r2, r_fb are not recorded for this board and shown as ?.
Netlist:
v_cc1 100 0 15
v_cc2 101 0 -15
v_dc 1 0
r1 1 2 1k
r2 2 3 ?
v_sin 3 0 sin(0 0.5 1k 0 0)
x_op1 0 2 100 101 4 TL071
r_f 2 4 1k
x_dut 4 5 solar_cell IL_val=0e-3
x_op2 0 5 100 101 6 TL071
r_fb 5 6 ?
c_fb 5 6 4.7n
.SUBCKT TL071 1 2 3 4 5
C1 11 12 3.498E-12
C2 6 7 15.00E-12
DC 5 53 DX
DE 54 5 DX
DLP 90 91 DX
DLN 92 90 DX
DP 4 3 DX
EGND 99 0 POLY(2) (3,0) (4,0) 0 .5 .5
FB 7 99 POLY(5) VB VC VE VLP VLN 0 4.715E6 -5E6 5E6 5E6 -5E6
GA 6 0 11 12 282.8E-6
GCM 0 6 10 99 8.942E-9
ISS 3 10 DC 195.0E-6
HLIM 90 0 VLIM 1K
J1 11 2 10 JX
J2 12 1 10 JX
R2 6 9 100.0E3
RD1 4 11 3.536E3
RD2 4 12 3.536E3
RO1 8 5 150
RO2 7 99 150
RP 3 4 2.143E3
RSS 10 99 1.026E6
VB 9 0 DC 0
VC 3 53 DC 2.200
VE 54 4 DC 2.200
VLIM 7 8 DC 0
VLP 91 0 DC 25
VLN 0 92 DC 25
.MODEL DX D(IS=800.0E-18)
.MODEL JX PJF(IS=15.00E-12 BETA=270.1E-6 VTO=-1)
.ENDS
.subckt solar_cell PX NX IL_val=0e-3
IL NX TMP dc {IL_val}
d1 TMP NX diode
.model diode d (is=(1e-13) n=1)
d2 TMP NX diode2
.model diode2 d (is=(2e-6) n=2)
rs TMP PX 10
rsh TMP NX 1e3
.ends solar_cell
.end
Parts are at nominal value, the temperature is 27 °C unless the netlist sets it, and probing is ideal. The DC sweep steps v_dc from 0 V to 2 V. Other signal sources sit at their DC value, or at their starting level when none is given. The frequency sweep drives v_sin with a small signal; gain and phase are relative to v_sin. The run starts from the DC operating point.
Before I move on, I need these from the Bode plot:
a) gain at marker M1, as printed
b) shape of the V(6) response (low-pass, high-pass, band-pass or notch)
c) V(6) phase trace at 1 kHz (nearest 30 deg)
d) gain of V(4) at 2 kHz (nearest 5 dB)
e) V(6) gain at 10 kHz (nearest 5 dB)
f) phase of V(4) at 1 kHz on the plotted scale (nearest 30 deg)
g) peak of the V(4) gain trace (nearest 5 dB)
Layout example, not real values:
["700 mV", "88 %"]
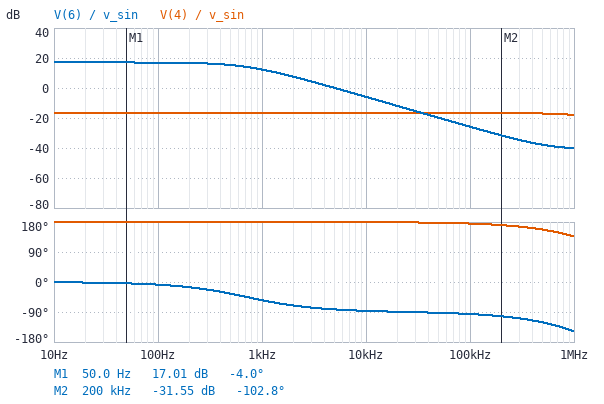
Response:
["17.01 dB", "low-pass", "-60 deg", "-15 dB", "-5 dB", "180 deg", "-15 dB"]
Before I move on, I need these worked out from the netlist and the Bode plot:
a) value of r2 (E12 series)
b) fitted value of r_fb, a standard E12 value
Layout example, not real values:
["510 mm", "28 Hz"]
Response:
["6.8 kΩ", "47 kΩ"]
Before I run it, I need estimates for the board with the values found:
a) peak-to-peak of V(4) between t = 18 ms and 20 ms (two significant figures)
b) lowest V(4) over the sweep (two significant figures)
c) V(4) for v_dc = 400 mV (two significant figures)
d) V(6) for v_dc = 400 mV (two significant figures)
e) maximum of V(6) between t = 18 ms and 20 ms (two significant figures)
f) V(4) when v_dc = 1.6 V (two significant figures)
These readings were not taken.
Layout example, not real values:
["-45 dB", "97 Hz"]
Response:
["150 mV", "-2.0 V", "-400 mV", "13 V", "2.0 V", "-1.6 V"]
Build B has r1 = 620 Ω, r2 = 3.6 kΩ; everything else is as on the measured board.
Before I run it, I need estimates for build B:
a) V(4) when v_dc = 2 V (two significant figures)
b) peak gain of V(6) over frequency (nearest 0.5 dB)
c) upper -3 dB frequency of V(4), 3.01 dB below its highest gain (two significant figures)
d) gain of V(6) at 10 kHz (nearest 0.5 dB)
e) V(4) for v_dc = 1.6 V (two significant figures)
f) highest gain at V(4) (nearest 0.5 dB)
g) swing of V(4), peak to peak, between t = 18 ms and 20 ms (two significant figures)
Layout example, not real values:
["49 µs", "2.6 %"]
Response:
["-3.2 V", "22.5 dB", "1.1 MHz", "-0.5 dB", "-2.6 V", "-11.0 dB", "280 mV"]
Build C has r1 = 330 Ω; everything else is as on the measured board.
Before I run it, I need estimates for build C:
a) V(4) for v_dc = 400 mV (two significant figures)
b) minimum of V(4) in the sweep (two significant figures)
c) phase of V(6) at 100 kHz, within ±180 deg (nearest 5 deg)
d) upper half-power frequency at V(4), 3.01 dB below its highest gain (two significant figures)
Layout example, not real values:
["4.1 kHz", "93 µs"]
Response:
["-1.2 V", "-6.1 V", "-100 deg", "730 kHz"]
